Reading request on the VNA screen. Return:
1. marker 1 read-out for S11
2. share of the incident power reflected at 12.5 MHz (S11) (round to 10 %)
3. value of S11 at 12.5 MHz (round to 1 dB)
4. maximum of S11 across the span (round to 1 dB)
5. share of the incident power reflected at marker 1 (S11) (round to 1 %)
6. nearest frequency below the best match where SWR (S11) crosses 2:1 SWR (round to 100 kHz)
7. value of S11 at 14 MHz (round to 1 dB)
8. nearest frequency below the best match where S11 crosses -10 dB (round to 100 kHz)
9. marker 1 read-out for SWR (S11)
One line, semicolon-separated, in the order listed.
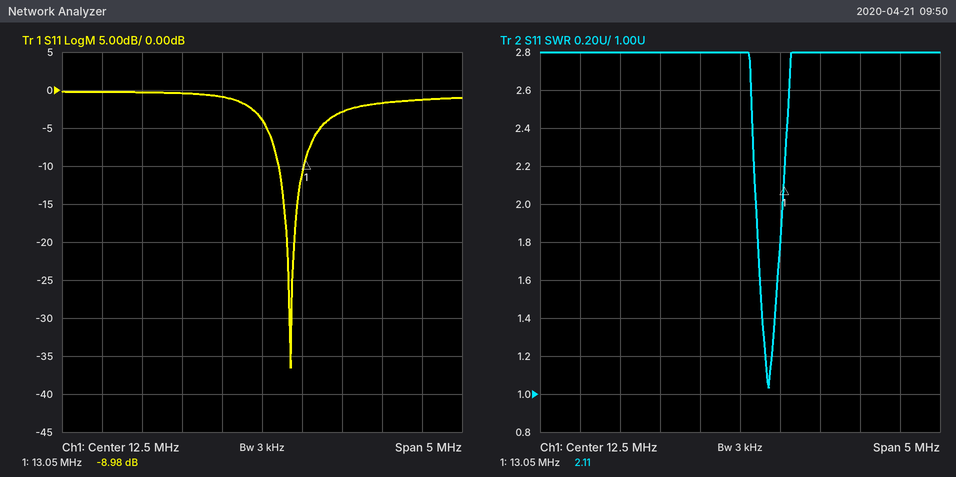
-8.98 dB; 40 %; -4 dB; 0 dB; 13 %; 12.7 MHz; -2 dB; 12.7 MHz; 2.11
